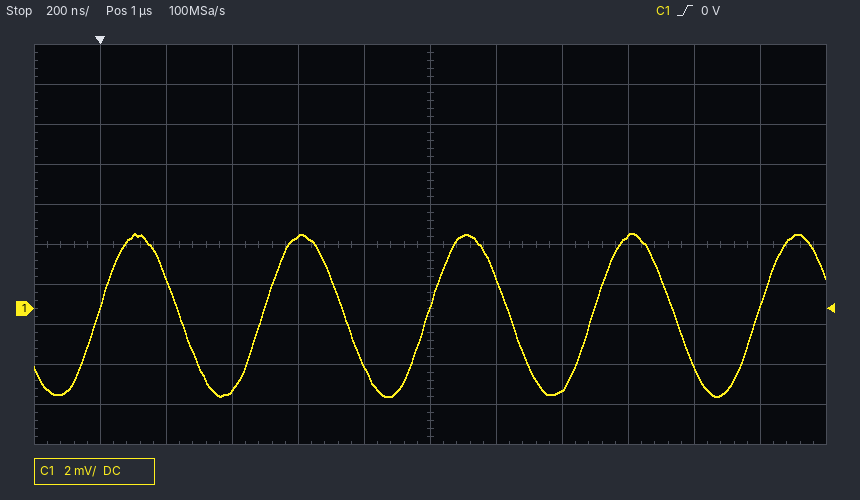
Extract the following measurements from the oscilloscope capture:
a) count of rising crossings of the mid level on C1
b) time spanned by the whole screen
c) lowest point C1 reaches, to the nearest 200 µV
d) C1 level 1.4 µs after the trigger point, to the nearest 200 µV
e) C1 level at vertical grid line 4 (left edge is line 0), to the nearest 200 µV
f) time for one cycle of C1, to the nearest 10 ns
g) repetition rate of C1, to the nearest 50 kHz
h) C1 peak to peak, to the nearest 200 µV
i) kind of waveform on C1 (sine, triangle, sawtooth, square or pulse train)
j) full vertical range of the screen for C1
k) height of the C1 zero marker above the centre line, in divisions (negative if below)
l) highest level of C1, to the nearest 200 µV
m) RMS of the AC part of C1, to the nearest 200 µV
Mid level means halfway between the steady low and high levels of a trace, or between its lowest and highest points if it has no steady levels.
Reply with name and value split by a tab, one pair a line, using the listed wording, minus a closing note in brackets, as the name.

count of rising crossings of the mid level on C1	5
time spanned by the whole screen	2.4 µs
lowest point C1 reaches, to the nearest 200 µV	-4.4 mV
C1 level 1.4 µs after the trigger point, to the nearest 200 µV	-4.0 mV
C1 level at vertical grid line 4 (left edge is line 0), to the nearest 200 µV	3.6 mV
time for one cycle of C1, to the nearest 10 ns	500 ns
repetition rate of C1, to the nearest 50 kHz	2.00 MHz
C1 peak to peak, to the nearest 200 µV	8.2 mV
kind of waveform on C1	sine
full vertical range of the screen for C1	20 mV
height of the C1 zero marker above the centre line, in divisions	-1.6 div
highest level of C1, to the nearest 200 µV	3.8 mV
RMS of the AC part of C1, to the nearest 200 µV	2.8 mV
